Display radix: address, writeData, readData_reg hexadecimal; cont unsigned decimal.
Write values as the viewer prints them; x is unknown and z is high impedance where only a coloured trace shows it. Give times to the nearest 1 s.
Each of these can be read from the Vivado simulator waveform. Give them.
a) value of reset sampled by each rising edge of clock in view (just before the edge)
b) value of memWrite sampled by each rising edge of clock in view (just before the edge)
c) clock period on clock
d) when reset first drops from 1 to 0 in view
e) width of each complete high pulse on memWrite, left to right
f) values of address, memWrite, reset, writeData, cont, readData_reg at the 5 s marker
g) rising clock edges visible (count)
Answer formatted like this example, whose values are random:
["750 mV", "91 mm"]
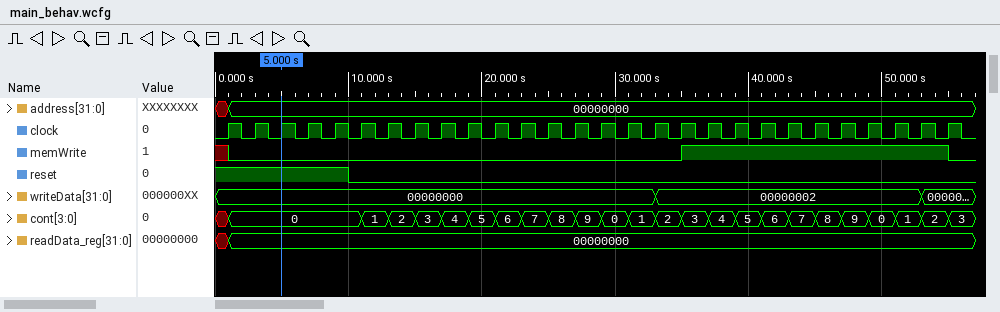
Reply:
["1 1 1 1 1 0 0 0 0 0 0 0 0 0 0 0 0 0 0 0 0 0 0 0 0 0 0 0", "x 0 0 0 0 0 0 0 0 0 0 0 0 0 0 0 0 0 1 1 1 1 1 1 1 1 1 1", "2 s", "10 s", "20 s", "address=00000000, memWrite=0, reset=1, writeData=00000000, cont=0, readData_reg=00000000", "28"]
